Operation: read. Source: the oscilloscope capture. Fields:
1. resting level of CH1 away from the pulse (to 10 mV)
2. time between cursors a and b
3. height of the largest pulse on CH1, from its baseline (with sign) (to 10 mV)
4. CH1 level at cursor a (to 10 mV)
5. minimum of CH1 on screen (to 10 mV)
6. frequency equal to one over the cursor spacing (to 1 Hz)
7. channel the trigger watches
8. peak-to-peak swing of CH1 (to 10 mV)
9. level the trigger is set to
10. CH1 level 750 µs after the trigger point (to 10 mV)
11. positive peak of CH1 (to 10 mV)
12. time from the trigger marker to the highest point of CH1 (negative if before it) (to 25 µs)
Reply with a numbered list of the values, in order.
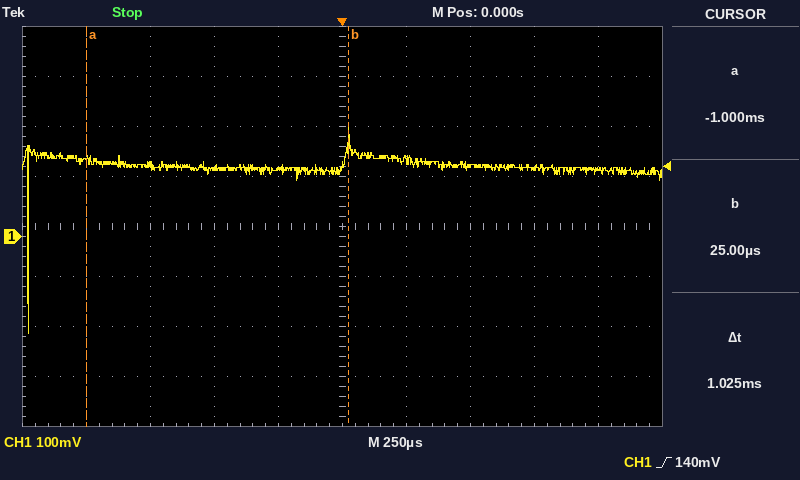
1. 140 mV
2. 1.025 ms
3. -330 mV
4. 150 mV
5. -190 mV
6. 976 Hz
7. CH1
8. 410 mV
9. 140 mV
10. 140 mV
11. 220 mV
12. +25 µs
